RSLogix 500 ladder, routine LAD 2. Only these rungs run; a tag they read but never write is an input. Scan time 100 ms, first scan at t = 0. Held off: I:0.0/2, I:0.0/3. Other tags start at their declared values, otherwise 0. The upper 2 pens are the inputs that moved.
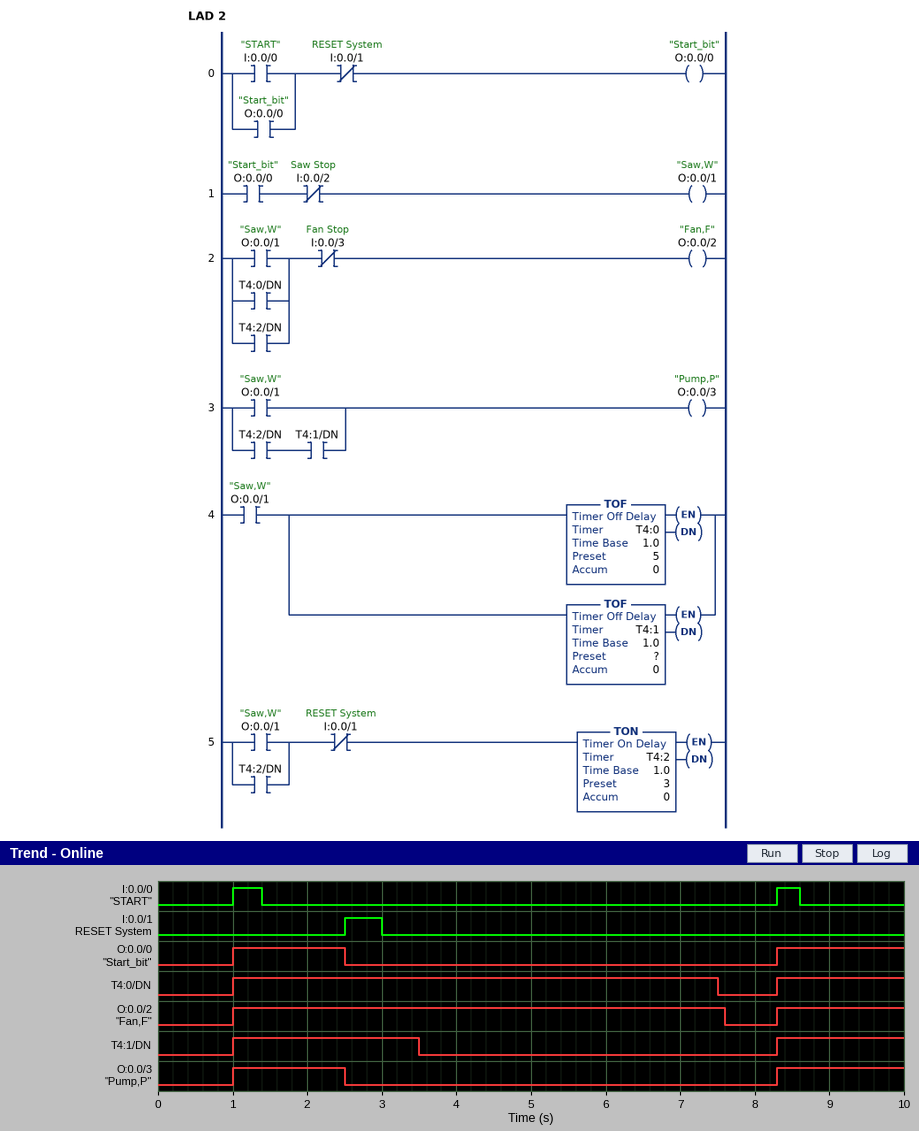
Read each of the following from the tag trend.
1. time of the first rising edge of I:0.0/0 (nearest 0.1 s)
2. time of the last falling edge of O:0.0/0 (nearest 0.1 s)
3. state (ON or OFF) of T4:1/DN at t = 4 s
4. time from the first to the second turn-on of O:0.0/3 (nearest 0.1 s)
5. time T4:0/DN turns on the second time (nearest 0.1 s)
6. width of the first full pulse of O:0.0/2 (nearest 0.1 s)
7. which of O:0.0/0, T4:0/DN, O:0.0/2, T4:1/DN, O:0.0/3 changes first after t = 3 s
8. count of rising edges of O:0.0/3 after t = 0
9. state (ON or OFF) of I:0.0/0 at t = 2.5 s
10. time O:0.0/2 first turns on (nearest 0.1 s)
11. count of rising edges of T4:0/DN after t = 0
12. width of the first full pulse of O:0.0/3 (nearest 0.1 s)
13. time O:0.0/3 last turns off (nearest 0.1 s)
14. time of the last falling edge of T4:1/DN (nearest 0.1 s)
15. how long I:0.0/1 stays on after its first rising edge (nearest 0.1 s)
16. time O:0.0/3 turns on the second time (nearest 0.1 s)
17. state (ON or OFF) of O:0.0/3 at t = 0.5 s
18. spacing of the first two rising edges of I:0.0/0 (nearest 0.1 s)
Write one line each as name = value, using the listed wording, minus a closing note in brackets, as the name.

time of the first rising edge of I:0.0/0 = 1.0 s
time of the last falling edge of O:0.0/0 = 2.5 s
state (ON or OFF) of T4:1/DN at t = 4 s = OFF
time from the first to the second turn-on of O:0.0/3 = 7.3 s
time T4:0/DN turns on the second time = 8.3 s
width of the first full pulse of O:0.0/2 = 6.6 s
which of O:0.0/0, T4:0/DN, O:0.0/2, T4:1/DN, O:0.0/3 changes first after t = 3 s = T4:1/DN
count of rising edges of O:0.0/3 after t = 0 = 2
state (ON or OFF) of I:0.0/0 at t = 2.5 s = OFF
time O:0.0/2 first turns on = 1.0 s
count of rising edges of T4:0/DN after t = 0 = 2
width of the first full pulse of O:0.0/3 = 1.5 s
time O:0.0/3 last turns off = 2.5 s
time of the last falling edge of T4:1/DN = 3.5 s
how long I:0.0/1 stays on after its first rising edge = 0.5 s
time O:0.0/3 turns on the second time = 8.3 s
state (ON or OFF) of O:0.0/3 at t = 0.5 s = OFF
spacing of the first two rising edges of I:0.0/0 = 7.3 s
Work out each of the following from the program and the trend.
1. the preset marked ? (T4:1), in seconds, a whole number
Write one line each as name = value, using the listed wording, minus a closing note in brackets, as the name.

the preset marked ? (T4:1), in seconds, a whole number = 1 s
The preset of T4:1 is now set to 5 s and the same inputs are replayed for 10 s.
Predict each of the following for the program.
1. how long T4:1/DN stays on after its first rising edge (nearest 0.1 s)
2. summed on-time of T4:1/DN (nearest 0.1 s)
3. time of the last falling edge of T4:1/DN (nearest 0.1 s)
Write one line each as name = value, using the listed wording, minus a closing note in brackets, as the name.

how long T4:1/DN stays on after its first rising edge = 6.5 s
summed on-time of T4:1/DN = 8.2 s
time of the last falling edge of T4:1/DN = 7.5 s
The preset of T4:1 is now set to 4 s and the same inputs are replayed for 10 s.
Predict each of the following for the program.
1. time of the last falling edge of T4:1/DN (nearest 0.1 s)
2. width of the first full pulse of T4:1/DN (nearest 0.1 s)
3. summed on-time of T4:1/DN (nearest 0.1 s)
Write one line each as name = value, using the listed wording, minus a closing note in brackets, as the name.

time of the last falling edge of T4:1/DN = 6.5 s
width of the first full pulse of T4:1/DN = 5.5 s
summed on-time of T4:1/DN = 7.2 s
